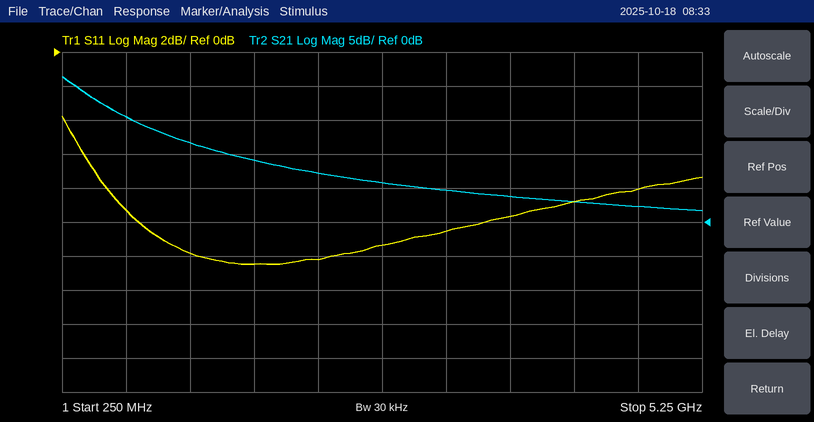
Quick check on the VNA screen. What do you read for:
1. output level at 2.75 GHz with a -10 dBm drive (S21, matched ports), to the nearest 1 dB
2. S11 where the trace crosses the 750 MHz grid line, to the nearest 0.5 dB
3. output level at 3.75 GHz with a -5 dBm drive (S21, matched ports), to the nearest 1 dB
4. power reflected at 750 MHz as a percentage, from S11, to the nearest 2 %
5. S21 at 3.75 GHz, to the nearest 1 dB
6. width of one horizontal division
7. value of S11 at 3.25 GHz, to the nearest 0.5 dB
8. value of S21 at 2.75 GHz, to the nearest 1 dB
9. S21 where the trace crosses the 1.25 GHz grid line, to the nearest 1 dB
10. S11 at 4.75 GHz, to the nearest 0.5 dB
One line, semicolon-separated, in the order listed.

-4 dBm; -9.5 dB; -1 dBm; 12 %; 4 dB; 500 MHz; -10.5 dB; 6 dB; 12 dB; -8.0 dB
